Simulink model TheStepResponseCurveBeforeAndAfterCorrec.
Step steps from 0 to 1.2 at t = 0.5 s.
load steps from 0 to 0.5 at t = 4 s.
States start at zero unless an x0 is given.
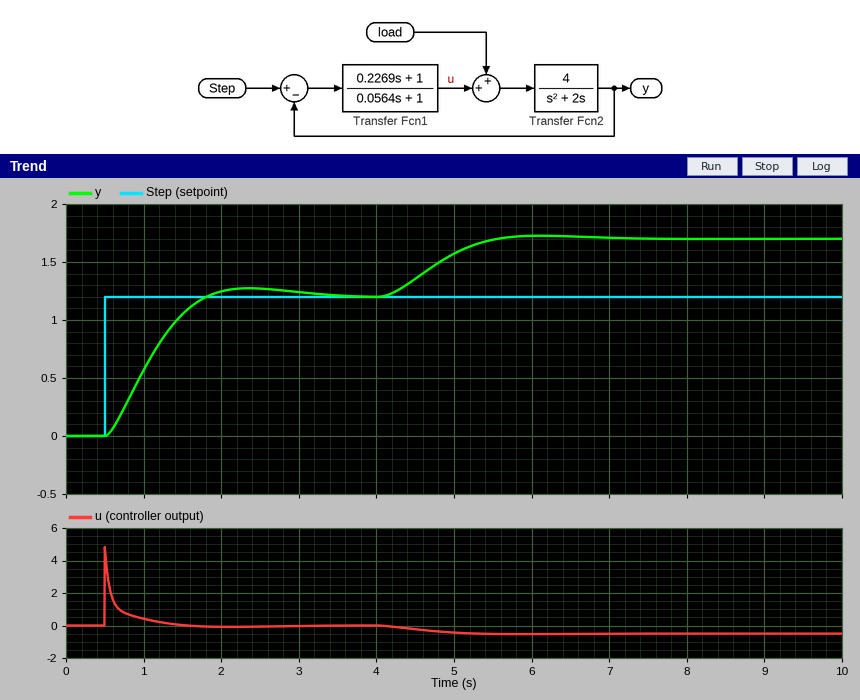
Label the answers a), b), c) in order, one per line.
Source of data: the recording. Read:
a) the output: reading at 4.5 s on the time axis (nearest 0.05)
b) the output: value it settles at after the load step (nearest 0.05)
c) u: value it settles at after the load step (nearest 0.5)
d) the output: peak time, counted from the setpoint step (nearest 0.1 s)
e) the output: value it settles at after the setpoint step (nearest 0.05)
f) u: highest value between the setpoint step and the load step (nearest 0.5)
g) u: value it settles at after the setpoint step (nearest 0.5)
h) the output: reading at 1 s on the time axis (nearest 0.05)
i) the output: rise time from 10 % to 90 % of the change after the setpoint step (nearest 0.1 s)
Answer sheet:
a) 1.35
b) 1.70
c) -0.5
d) 1.9 s
e) 1.20
f) 5.0
g) 0.0
h) 0.55
i) 0.9 s
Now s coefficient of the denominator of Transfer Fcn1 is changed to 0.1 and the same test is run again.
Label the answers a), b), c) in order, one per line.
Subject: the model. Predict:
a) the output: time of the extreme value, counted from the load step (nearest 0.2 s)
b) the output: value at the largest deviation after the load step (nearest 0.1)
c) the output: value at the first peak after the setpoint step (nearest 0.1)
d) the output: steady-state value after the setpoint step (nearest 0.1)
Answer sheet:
a) 2.0 s
b) 1.7
c) 1.3
d) 1.2
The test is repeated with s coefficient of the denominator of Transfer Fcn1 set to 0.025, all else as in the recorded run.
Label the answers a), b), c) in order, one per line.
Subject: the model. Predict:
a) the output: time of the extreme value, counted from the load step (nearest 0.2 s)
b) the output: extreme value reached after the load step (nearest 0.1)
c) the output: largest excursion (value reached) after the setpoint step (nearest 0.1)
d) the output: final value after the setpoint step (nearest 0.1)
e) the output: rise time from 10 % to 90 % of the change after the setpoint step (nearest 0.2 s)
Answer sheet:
a) 2.2 s
b) 1.7
c) 1.3
d) 1.2
e) 1.0 s
